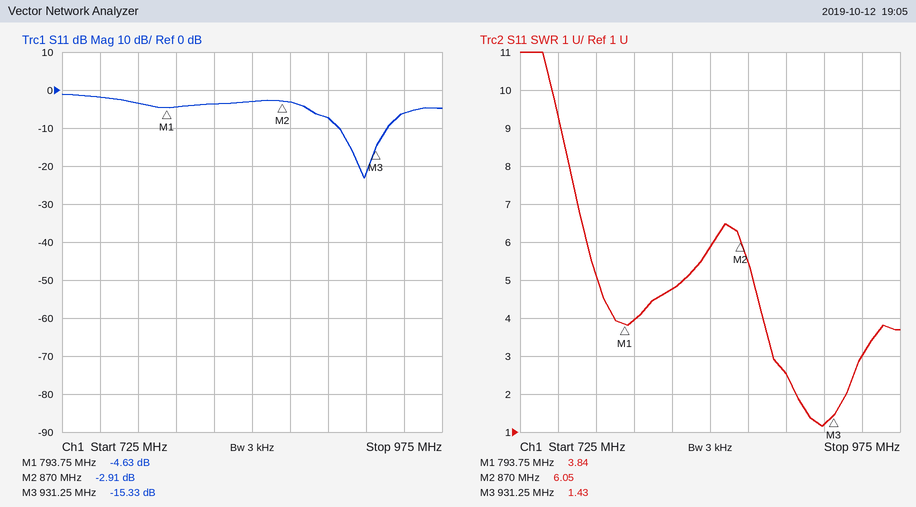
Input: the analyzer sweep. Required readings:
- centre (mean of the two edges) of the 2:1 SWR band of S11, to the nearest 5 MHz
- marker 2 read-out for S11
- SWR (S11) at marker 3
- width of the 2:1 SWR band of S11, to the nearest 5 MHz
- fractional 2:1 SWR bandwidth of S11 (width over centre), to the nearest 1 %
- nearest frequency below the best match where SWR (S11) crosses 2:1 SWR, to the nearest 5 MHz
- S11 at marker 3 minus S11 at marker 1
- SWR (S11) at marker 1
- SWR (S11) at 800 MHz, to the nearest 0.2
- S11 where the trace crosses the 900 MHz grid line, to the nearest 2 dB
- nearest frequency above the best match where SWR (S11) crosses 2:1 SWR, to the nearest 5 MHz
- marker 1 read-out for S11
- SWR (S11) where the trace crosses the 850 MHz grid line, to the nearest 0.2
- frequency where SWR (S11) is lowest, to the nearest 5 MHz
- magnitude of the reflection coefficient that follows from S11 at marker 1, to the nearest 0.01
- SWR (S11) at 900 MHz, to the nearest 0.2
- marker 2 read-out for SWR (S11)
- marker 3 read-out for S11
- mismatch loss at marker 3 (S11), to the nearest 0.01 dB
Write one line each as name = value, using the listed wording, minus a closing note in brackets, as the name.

centre (mean of the two edges) of the 2:1 SWR band of S11, to the nearest 5 MHz = 925 MHz
marker 2 read-out for S11 = -2.91 dB
SWR (S11) at marker 3 = 1.43
width of the 2:1 SWR band of S11, to the nearest 5 MHz = 35 MHz
fractional 2:1 SWR bandwidth of S11 (width over centre), to the nearest 1 % = 4 %
nearest frequency below the best match where SWR (S11) crosses 2:1 SWR, to the nearest 5 MHz = 905 MHz
S11 at marker 3 minus S11 at marker 1 = -10.70 dB
SWR (S11) at marker 1 = 3.84
SWR (S11) at 800 MHz, to the nearest 0.2 = 4.0
S11 where the trace crosses the 900 MHz grid line, to the nearest 2 dB = -8 dB
nearest frequency above the best match where SWR (S11) crosses 2:1 SWR, to the nearest 5 MHz = 940 MHz
marker 1 read-out for S11 = -4.63 dB
SWR (S11) where the trace crosses the 850 MHz grid line, to the nearest 0.2 = 5.8
frequency where SWR (S11) is lowest, to the nearest 5 MHz = 925 MHz
magnitude of the reflection coefficient that follows from S11 at marker 1, to the nearest 0.01 = 0.59
SWR (S11) at 900 MHz, to the nearest 0.2 = 2.6
marker 2 read-out for SWR = 6.05
marker 3 read-out for S11 = -15.33 dB
mismatch loss at marker 3 (S11), to the nearest 0.01 dB = 0.13 dB
